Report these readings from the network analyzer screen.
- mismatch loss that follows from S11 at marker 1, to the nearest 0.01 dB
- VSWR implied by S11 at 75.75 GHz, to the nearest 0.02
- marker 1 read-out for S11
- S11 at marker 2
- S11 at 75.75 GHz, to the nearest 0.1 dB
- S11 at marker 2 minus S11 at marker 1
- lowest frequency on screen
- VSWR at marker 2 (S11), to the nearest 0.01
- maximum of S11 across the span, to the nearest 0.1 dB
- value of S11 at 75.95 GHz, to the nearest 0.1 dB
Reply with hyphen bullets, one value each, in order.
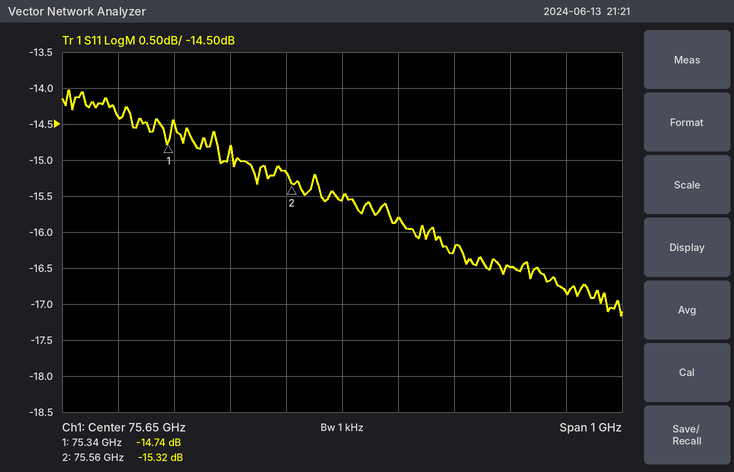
- 0.15 dB
- 1.38
- -14.74 dB
- -15.32 dB
- -15.8 dB
- -0.58 dB
- 75.15 GHz
- 1.41
- -14.0 dB
- -16.5 dB
